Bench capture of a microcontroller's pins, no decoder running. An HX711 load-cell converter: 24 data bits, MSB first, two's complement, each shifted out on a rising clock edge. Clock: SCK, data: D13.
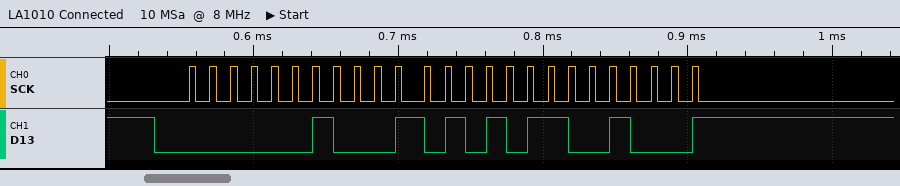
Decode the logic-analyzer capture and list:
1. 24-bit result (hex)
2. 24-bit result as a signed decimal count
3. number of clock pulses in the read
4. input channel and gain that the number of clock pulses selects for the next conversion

0x022AC8
142024
25
channel A, gain 128
